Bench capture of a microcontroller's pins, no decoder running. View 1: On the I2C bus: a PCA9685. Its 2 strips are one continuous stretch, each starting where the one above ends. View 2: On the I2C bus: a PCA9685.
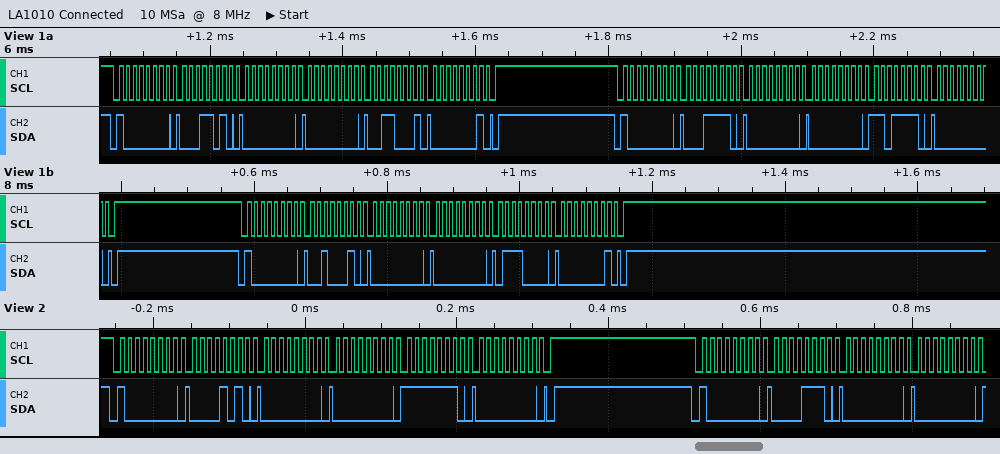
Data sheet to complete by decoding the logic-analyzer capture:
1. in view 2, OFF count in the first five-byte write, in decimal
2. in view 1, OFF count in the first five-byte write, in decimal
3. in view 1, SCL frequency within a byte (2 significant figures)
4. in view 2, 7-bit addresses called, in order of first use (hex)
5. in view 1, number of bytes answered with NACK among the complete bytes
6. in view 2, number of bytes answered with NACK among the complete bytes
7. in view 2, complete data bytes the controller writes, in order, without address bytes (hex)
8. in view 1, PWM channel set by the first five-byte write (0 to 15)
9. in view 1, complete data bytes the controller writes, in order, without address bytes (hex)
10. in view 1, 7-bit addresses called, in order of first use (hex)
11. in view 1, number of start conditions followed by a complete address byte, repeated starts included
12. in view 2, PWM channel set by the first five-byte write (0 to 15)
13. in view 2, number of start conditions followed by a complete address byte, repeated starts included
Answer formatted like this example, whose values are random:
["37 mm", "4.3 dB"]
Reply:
["254", "305", "100 kHz", "0x40", "0", "0", "0A 00 00 FE 00 0E 00 00", "5", "1A 00 00 31 01 1E 00 00 DE 00 22 00 00 70 01", "0x40", "3", "1", "2"]
